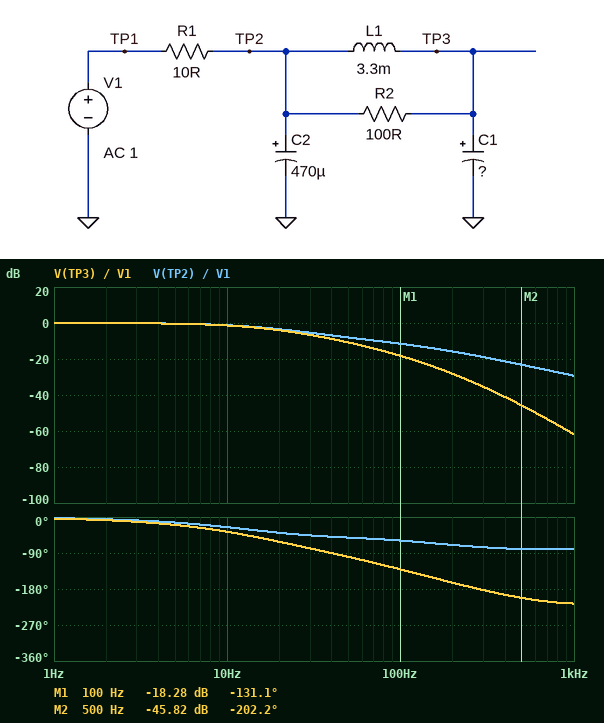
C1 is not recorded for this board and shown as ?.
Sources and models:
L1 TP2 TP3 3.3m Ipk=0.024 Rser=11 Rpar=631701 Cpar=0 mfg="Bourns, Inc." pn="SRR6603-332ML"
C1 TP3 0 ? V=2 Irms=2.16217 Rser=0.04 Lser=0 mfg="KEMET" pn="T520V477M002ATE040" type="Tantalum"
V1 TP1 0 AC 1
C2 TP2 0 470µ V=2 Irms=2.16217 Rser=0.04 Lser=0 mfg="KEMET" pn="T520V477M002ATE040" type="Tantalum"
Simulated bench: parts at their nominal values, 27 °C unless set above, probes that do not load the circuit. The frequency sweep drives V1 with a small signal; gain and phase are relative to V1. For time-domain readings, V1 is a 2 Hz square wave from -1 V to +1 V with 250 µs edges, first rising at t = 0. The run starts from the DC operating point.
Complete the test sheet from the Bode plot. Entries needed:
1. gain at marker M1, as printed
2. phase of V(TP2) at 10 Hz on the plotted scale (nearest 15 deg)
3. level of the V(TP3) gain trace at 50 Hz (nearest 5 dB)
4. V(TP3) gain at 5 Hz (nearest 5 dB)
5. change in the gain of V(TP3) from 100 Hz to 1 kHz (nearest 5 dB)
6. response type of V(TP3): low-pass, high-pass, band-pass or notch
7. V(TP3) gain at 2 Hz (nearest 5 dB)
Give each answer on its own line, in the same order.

-18.28 dB
-30 deg
-10 dB
0 dB
-45 dB
low-pass
0 dB
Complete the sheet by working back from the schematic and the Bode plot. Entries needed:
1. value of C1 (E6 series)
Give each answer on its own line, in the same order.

330 µF
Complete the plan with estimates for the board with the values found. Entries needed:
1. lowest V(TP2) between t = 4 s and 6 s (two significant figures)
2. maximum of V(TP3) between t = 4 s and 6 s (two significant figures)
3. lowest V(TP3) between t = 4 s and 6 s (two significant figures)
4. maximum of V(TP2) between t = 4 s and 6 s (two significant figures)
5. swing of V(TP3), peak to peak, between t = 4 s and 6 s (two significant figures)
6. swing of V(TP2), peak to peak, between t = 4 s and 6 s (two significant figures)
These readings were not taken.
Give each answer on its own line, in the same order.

-1.0 V
1.0 V
-1.0 V
1.0 V
2.0 V
2.0 V
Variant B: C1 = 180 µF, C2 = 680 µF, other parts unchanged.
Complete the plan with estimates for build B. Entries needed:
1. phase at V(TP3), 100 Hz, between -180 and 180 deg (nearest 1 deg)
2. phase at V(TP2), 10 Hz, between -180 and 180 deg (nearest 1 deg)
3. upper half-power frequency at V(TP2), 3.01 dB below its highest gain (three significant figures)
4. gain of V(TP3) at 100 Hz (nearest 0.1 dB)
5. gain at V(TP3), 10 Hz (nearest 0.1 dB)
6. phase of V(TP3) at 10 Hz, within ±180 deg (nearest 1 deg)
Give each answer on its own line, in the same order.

-124 deg
-28 deg
17.8 Hz
-16.9 dB
-1.2 dB
-34 deg
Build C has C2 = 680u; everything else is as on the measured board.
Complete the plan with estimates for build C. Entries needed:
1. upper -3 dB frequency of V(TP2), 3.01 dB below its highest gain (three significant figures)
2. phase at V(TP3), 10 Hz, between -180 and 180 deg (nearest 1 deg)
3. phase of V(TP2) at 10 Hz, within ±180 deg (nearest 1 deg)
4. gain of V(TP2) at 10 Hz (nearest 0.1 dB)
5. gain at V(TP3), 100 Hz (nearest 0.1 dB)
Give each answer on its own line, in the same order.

14.6 Hz
-43 deg
-31 deg
-1.7 dB
-20.7 dB
